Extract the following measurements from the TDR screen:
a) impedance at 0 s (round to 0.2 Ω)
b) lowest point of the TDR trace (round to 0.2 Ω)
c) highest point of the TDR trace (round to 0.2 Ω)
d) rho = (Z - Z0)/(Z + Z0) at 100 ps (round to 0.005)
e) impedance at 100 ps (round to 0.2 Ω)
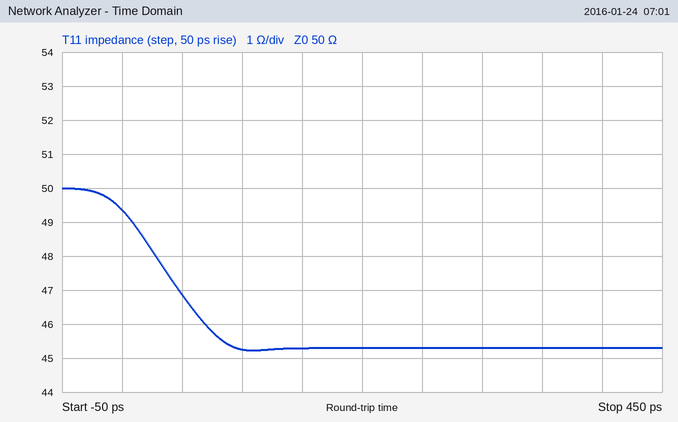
49.4 Ω
45.2 Ω
50.0 Ω
-0.050
45.2 Ω
